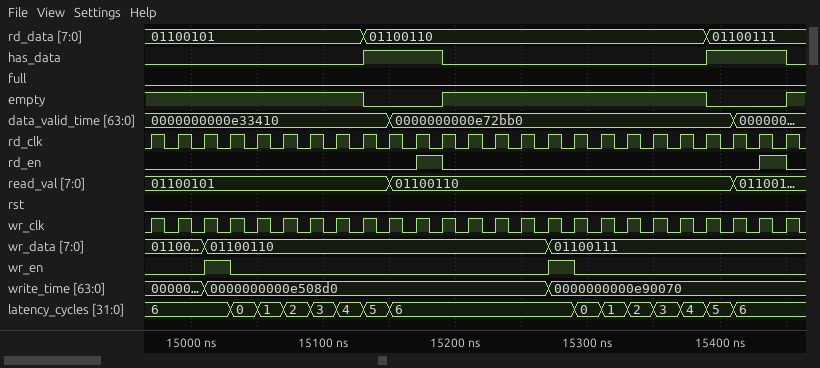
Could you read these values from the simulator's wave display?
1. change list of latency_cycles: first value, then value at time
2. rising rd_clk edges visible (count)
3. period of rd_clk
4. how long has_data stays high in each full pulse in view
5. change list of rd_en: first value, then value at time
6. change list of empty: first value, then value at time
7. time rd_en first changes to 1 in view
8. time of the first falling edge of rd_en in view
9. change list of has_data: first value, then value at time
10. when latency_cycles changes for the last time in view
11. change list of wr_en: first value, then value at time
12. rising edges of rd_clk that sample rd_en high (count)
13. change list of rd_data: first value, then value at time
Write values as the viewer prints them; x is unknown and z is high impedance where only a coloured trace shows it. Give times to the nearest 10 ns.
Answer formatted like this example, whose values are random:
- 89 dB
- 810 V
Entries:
- 6, 0 at 15030 ns, 1 at 15050 ns, 2 at 15070 ns, 3 at 15090 ns, 4 at 15110 ns, 5 at 15130 ns, 6 at 15150 ns, 0 at 15290 ns, 1 at 15310 ns, 2 at 15330 ns, 3 at 15350 ns, 4 at 15370 ns, 5 at 15390 ns, 6 at 15410 ns
- 25
- 20 ns
- 60 ns, 60 ns
- 0, 1 at 15170 ns, 0 at 15190 ns, 1 at 15430 ns, 0 at 15450 ns
- 1, 0 at 15130 ns, 1 at 15190 ns, 0 at 15390 ns, 1 at 15450 ns
- 15170 ns
- 15190 ns
- 0, 1 at 15130 ns, 0 at 15190 ns, 1 at 15390 ns, 0 at 15450 ns
- 15410 ns
- 0, 1 at 15010 ns, 0 at 15030 ns, 1 at 15270 ns, 0 at 15290 ns
- 2
- 01100101, 01100110 at 15130 ns, 01100111 at 15390 ns
